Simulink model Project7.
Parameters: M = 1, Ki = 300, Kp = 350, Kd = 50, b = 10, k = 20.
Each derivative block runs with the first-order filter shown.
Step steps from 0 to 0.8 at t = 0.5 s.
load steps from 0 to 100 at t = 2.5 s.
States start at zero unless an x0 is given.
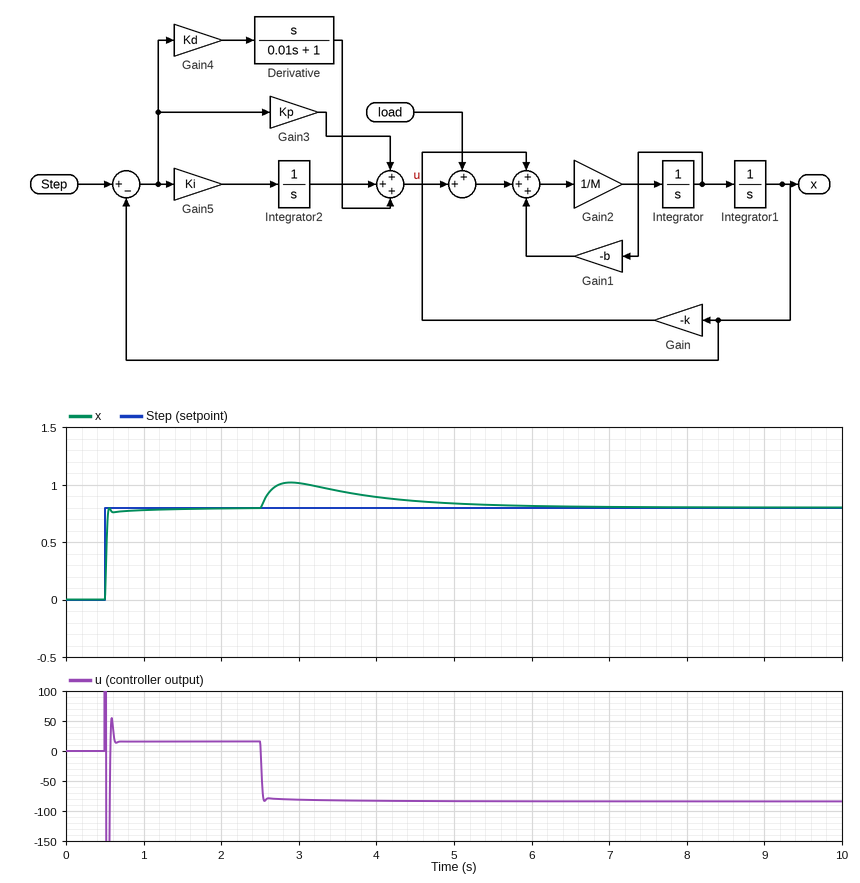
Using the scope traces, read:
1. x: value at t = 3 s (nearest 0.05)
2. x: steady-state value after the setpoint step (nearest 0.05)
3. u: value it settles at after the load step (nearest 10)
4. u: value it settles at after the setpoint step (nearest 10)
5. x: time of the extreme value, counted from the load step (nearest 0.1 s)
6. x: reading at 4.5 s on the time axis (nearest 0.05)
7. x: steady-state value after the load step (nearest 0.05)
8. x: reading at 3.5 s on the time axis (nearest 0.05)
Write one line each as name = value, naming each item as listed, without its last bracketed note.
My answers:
x: value at t = 3 s = 1.00
x: steady-state value after the setpoint step = 0.80
u: value it settles at after the load step = -80
u: value it settles at after the setpoint step = 20
x: time of the extreme value, counted from the load step = 0.4 s
x: reading at 4.5 s on the time axis = 0.85
x: steady-state value after the load step = 0.80
x: reading at 3.5 s on the time axis = 0.95
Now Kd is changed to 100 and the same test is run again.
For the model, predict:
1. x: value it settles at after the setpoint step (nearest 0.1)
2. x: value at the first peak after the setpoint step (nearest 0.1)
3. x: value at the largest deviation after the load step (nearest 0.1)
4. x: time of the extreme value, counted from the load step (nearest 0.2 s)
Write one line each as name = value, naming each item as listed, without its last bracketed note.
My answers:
x: value it settles at after the setpoint step = 0.8
x: value at the first peak after the setpoint step = 0.9
x: value at the largest deviation after the load step = 1.0
x: time of the extreme value, counted from the load step = 0.6 s
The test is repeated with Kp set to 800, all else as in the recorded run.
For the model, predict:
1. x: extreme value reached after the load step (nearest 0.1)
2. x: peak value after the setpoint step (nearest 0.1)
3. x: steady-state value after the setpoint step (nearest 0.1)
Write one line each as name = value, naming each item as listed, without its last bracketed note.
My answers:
x: extreme value reached after the load step = 0.9
x: peak value after the setpoint step = 0.9
x: steady-state value after the setpoint step = 0.8
